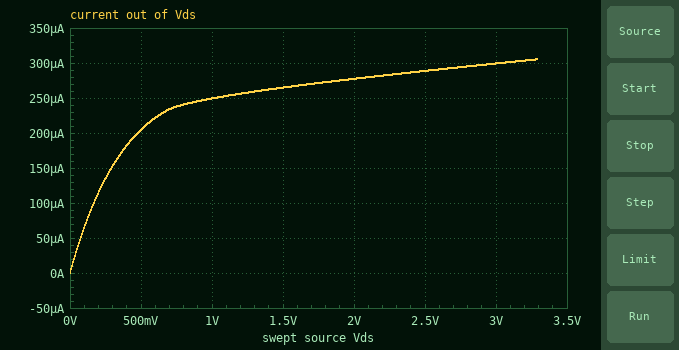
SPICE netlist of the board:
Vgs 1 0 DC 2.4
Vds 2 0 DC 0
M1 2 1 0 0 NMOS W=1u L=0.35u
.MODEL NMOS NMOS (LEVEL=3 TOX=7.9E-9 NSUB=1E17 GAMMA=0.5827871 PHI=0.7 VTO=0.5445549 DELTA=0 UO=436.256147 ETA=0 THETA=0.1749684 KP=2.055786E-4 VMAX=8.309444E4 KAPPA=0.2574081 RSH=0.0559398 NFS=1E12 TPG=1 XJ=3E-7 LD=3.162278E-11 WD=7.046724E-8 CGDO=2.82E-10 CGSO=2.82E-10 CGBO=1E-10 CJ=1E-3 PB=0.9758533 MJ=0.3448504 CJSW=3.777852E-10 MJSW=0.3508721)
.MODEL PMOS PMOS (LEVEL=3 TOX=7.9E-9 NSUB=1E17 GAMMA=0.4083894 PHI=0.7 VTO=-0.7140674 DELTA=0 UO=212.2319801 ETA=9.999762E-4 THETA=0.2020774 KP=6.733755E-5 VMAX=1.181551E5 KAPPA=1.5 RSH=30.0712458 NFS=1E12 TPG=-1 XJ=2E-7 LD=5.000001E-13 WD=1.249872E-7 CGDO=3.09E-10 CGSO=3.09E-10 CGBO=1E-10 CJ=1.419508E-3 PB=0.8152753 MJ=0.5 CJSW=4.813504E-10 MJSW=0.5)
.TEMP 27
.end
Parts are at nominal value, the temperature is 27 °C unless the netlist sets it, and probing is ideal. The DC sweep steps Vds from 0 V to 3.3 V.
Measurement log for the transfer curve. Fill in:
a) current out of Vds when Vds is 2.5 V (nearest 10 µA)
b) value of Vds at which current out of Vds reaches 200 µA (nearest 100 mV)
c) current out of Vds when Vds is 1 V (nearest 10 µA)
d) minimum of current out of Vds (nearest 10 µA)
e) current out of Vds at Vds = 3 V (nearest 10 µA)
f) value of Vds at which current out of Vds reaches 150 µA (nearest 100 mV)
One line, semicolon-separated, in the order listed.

290 µA; 500 mV; 250 µA; 0 A; 300 µA; 300 mV
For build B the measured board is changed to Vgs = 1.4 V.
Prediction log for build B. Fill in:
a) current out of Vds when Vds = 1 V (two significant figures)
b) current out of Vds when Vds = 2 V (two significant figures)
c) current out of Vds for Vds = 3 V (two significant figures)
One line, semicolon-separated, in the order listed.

100 µA; 110 µA; 120 µA
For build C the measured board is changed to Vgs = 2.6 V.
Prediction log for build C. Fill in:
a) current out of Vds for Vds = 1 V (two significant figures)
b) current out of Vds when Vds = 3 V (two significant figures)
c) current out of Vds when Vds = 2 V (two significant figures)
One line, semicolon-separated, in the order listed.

280 µA; 340 µA; 310 µA
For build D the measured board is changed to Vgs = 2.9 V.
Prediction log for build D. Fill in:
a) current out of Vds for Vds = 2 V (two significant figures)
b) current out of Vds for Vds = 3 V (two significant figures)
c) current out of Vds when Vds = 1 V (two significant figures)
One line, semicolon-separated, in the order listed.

360 µA; 390 µA; 320 µA
